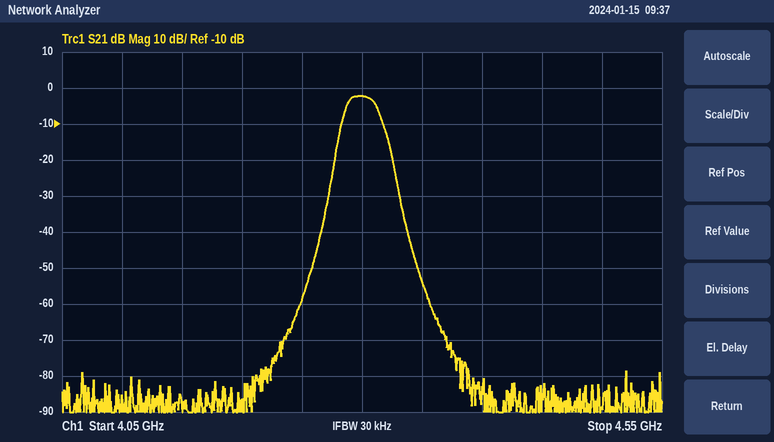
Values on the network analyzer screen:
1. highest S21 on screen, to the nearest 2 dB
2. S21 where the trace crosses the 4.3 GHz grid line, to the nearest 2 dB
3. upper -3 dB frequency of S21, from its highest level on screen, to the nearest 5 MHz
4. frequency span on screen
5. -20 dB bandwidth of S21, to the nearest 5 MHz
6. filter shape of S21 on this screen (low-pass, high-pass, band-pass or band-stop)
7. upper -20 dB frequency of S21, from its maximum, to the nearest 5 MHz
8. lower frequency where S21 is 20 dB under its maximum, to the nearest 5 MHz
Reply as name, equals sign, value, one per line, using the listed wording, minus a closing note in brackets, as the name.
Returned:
highest S21 on screen, to the nearest 2 dB = -2 dB
S21 where the trace crosses the 4.3 GHz grid line, to the nearest 2 dB = -2 dB
upper -3 dB frequency of S21, from its highest level on screen, to the nearest 5 MHz = 4.310 GHz
frequency span on screen = 500 MHz
-20 dB bandwidth of S21, to the nearest 5 MHz = 50 MHz
filter shape of S21 on this screen = band-pass
upper -20 dB frequency of S21, from its maximum, to the nearest 5 MHz = 4.325 GHz
lower frequency where S21 is 20 dB under its maximum, to the nearest 5 MHz = 4.275 GHz
